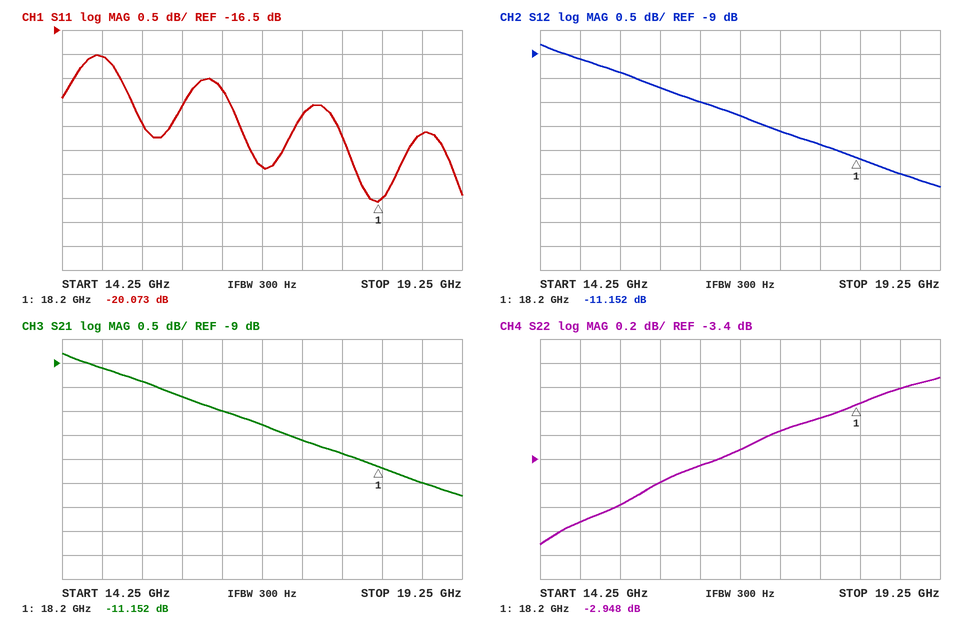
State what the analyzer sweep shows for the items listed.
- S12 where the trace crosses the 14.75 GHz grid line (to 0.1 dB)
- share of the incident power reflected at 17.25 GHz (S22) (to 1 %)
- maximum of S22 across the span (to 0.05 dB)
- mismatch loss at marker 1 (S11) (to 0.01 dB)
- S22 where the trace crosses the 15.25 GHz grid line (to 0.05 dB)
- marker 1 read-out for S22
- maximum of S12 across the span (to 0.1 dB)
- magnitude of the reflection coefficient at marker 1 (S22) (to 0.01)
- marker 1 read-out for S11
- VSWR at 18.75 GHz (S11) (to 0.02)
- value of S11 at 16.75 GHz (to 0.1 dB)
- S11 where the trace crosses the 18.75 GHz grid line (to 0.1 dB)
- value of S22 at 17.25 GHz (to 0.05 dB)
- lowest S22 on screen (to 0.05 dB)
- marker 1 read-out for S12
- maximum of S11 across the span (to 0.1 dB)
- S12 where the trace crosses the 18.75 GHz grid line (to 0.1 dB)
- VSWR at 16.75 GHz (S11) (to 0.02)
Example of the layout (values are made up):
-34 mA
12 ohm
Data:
-9.1 dB
48 %
-2.70 dB
0.04 dB
-3.80 dB
-2.948 dB
-8.8 dB
0.71
-20.073 dB
1.26
-19.3 dB
-18.7 dB
-3.15 dB
-4.10 dB
-11.152 dB
-17.0 dB
-11.5 dB
1.24
